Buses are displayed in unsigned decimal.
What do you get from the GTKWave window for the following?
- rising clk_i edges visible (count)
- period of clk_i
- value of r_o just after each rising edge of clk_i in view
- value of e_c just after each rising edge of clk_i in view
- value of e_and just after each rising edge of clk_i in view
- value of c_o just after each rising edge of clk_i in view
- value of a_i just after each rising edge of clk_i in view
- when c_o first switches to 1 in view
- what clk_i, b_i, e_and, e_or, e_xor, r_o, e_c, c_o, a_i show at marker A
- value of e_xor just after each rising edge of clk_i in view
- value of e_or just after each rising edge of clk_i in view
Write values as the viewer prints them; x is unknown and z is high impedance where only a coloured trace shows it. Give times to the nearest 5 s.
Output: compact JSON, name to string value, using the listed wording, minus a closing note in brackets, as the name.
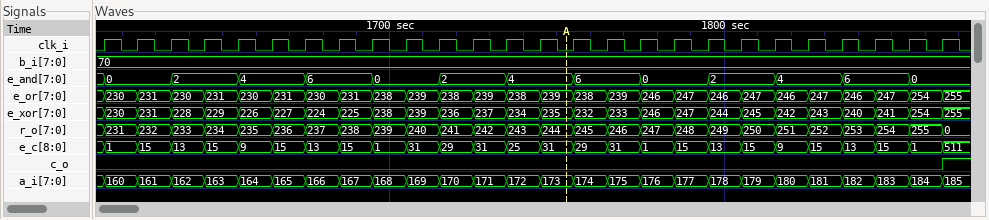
{"rising clk_i edges visible": "26", "period of clk_i": "10 s", "value of r_o just after each rising edge of clk_i in view": "231, 232, 233, 234, 235, 236, 237, 238, 239, 240, 241, 242, 243, 244, 245, 246, 247, 248, 249, 250, 251, 252, 253, 254, 255, 0", "value of e_c just after each rising edge of clk_i in view": "1, 15, 13, 15, 9, 15, 13, 15, 1, 31, 29, 31, 25, 31, 29, 31, 1, 15, 13, 15, 9, 15, 13, 15, 1, 511", "value of e_and just after each rising edge of clk_i in view": "0, 0, 2, 2, 4, 4, 6, 6, 0, 0, 2, 2, 4, 4, 6, 6, 0, 0, 2, 2, 4, 4, 6, 6, 0, 0", "value of c_o just after each rising edge of clk_i in view": "0 0 0 0 0 0 0 0 0 0 0 0 0 0 0 0 0 0 0 0 0 0 0 0 0 1", "value of a_i just after each rising edge of clk_i in view": "160, 161, 162, 163, 164, 165, 166, 167, 168, 169, 170, 171, 172, 173, 174, 175, 176, 177, 178, 179, 180, 181, 182, 183, 184, 185", "when c_o first switches to 1 in view": "1865 s", "what clk_i, b_i, e_and, e_or, e_xor, r_o, e_c, c_o, a_i show at marker A": "clk_i=0, b_i=70, e_and=4, e_or=239, e_xor=235, r_o=244, e_c=31, c_o=0, a_i=173", "value of e_xor just after each rising edge of clk_i in view": "230, 231, 228, 229, 226, 227, 224, 225, 238, 239, 236, 237, 234, 235, 232, 233, 246, 247, 244, 245, 242, 243, 240, 241, 254, 255", "value of e_or just after each rising edge of clk_i in view": "230, 231, 230, 231, 230, 231, 230, 231, 238, 239, 238, 239, 238, 239, 238, 239, 246, 247, 246, 247, 246, 247, 246, 247, 254, 255"}
